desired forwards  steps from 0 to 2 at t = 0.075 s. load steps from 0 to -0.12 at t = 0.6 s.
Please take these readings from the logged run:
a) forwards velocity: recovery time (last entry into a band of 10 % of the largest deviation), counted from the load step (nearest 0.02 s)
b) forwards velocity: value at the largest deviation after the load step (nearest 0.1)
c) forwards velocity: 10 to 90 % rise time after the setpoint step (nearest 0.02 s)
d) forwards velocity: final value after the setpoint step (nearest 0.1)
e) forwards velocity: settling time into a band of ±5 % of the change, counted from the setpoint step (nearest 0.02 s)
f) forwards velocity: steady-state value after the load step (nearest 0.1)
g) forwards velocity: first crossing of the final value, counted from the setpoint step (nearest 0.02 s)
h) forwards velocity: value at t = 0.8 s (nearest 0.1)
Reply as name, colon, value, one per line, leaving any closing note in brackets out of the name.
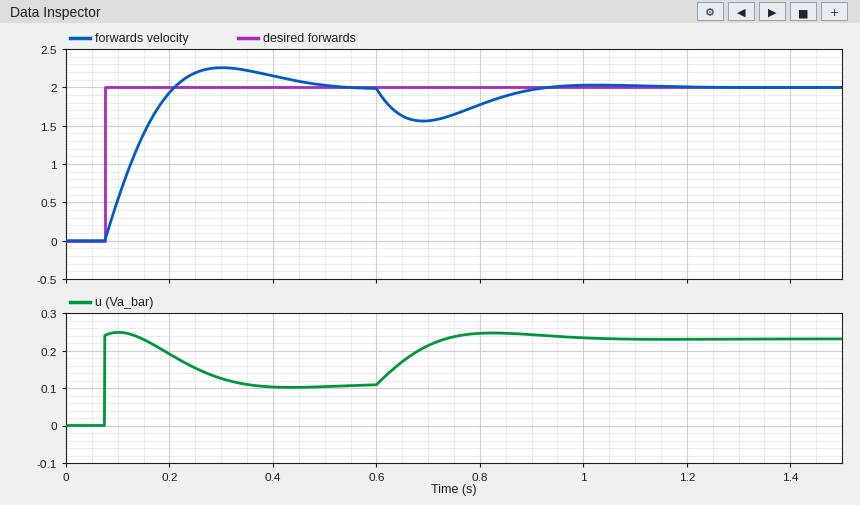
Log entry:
forwards velocity: recovery time (last entry into a band of 10 % of the largest deviation), counted from the load step: 0.30 s
forwards velocity: value at the largest deviation after the load step: 1.6
forwards velocity: 10 to 90 % rise time after the setpoint step: 0.10 s
forwards velocity: final value after the setpoint step: 2.0
forwards velocity: settling time into a band of ±5 % of the change, counted from the setpoint step: 0.36 s
forwards velocity: steady-state value after the load step: 2.0
forwards velocity: first crossing of the final value, counted from the setpoint step: 0.14 s
forwards velocity: value at t = 0.8 s: 1.8
